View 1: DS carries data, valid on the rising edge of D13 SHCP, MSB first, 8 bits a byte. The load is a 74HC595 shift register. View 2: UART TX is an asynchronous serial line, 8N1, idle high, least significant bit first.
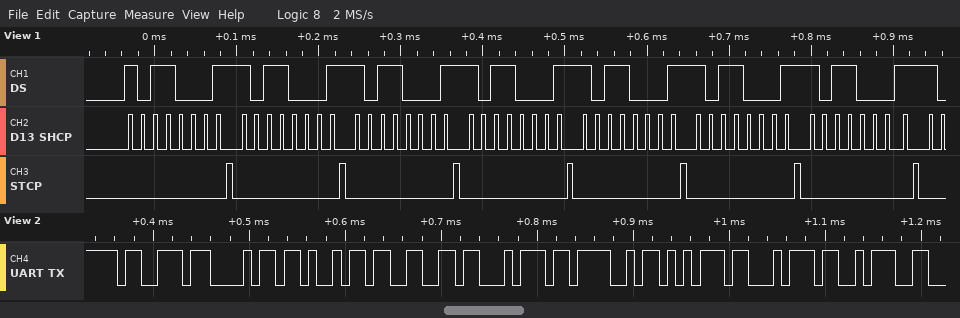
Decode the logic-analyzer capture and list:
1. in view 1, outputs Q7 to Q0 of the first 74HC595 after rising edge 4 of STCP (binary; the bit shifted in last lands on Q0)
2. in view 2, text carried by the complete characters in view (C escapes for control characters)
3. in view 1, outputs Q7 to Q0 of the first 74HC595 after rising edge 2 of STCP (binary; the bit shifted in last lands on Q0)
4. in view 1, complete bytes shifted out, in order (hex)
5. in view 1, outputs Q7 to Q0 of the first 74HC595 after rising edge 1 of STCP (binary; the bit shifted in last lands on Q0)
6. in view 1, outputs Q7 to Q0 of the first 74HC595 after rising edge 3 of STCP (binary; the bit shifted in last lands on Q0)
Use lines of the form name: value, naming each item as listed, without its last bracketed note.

in view 1, outputs Q7 to Q0 of the first 74HC595 after rising edge 4 of STCP: 10110001
in view 2, text carried by the complete characters in view: "shiftOut:"
in view 1, outputs Q7 to Q0 of the first 74HC595 after rising edge 2 of STCP: 10110001
in view 1, complete bytes shifted out, in order: B1 B1 B1 B1 B1 B1 B1
in view 1, outputs Q7 to Q0 of the first 74HC595 after rising edge 1 of STCP: 10110001
in view 1, outputs Q7 to Q0 of the first 74HC595 after rising edge 3 of STCP: 10110001
